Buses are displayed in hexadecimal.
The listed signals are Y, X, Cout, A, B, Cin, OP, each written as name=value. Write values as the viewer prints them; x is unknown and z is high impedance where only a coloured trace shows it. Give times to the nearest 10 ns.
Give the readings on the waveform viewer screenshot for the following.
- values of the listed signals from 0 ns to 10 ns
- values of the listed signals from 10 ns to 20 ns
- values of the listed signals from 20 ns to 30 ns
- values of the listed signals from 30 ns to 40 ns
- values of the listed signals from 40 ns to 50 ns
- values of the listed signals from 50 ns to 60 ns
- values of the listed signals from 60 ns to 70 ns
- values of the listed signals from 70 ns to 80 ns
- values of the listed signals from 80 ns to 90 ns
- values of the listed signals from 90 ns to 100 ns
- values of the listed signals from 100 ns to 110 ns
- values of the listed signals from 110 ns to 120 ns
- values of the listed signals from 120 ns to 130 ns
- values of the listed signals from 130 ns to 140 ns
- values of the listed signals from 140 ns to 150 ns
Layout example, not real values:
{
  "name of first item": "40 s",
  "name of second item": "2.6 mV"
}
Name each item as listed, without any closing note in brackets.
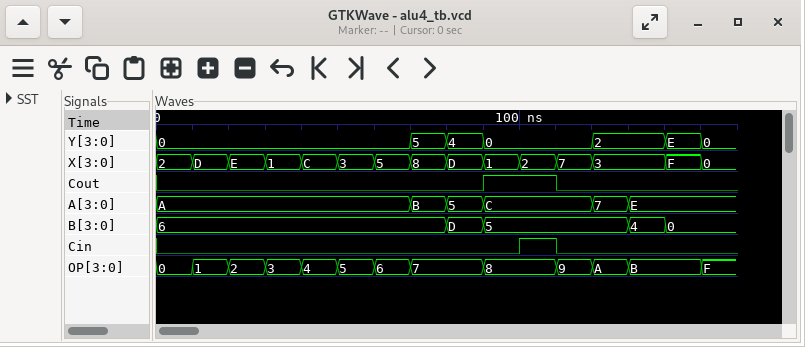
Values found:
{
  "values of the listed signals from 0 ns to 10 ns": "Y=0, X=2, Cout=0, A=A, B=6, Cin=0, OP=0",
  "values of the listed signals from 10 ns to 20 ns": "Y=0, X=D, Cout=0, A=A, B=6, Cin=0, OP=1",
  "values of the listed signals from 20 ns to 30 ns": "Y=0, X=E, Cout=0, A=A, B=6, Cin=0, OP=2",
  "values of the listed signals from 30 ns to 40 ns": "Y=0, X=1, Cout=0, A=A, B=6, Cin=0, OP=3",
  "values of the listed signals from 40 ns to 50 ns": "Y=0, X=C, Cout=0, A=A, B=6, Cin=0, OP=4",
  "values of the listed signals from 50 ns to 60 ns": "Y=0, X=3, Cout=0, A=A, B=6, Cin=0, OP=5",
  "values of the listed signals from 60 ns to 70 ns": "Y=0, X=5, Cout=0, A=A, B=6, Cin=0, OP=6",
  "values of the listed signals from 70 ns to 80 ns": "Y=5, X=8, Cout=0, A=B, B=6, Cin=0, OP=7",
  "values of the listed signals from 80 ns to 90 ns": "Y=4, X=D, Cout=0, A=5, B=D, Cin=0, OP=7",
  "values of the listed signals from 90 ns to 100 ns": "Y=0, X=1, Cout=1, A=C, B=5, Cin=0, OP=8",
  "values of the listed signals from 100 ns to 110 ns": "Y=0, X=2, Cout=1, A=C, B=5, Cin=1, OP=8",
  "values of the listed signals from 110 ns to 120 ns": "Y=0, X=7, Cout=0, A=C, B=5, Cin=0, OP=9",
  "values of the listed signals from 120 ns to 130 ns": "Y=2, X=3, Cout=0, A=7, B=5, Cin=0, OP=A",
  "values of the listed signals from 130 ns to 140 ns": "Y=2, X=3, Cout=0, A=E, B=4, Cin=0, OP=B",
  "values of the listed signals from 140 ns to 150 ns": "Y=E, X=F, Cout=0, A=E, B=0, Cin=0, OP=B"
}
